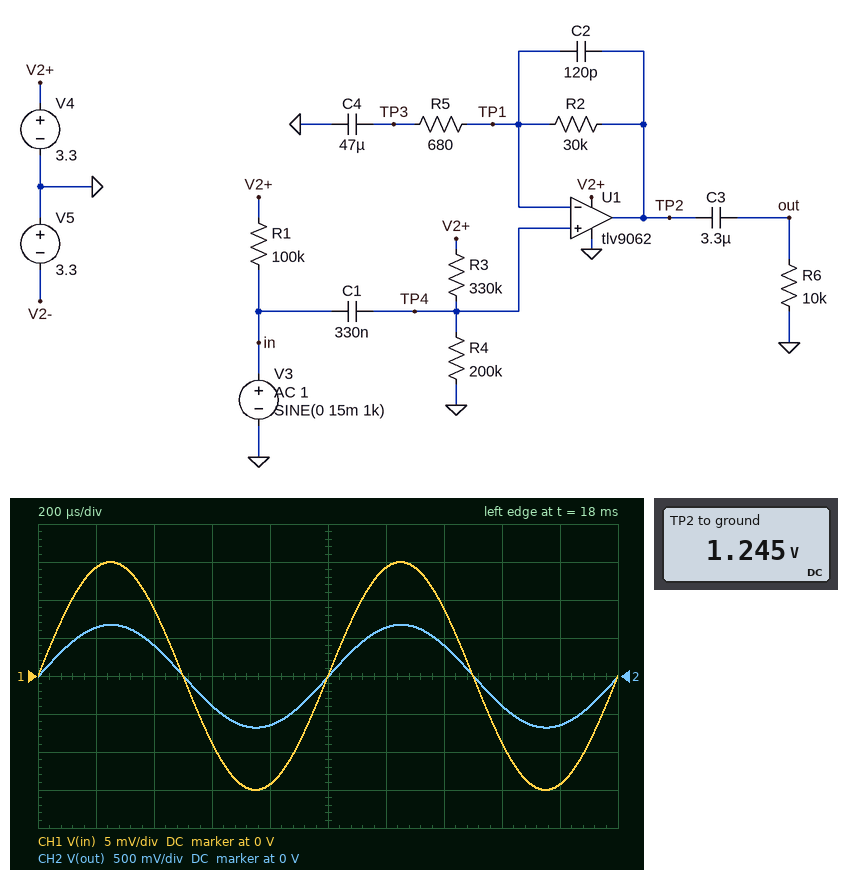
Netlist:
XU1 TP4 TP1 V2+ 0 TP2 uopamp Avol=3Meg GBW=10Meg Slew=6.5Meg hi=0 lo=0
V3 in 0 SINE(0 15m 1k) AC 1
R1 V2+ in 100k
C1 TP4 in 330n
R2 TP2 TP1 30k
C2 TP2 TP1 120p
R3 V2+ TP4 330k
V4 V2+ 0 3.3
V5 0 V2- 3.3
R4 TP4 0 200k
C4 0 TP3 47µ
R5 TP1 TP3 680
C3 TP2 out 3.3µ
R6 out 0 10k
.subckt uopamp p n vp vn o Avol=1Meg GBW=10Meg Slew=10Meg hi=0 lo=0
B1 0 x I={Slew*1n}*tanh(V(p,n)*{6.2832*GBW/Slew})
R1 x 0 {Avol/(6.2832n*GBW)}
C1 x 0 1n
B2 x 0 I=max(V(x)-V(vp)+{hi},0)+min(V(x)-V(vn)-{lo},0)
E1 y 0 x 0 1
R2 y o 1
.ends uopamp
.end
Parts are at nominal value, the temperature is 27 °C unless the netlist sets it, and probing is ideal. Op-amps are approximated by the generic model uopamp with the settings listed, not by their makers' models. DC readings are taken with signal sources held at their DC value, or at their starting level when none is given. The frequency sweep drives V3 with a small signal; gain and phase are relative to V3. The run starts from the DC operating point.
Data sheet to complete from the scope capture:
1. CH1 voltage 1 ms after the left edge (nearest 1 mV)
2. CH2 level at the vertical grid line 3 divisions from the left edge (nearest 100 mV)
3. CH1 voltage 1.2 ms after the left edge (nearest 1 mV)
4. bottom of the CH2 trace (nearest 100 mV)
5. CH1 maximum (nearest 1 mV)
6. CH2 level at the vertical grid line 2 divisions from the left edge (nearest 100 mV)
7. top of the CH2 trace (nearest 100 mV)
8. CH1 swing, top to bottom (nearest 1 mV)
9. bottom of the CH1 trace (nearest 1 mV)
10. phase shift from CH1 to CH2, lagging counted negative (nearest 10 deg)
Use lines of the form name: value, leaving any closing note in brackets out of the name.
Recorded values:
CH1 voltage 1 ms after the left edge: 0 V
CH2 level at the vertical grid line 3 divisions from the left edge: -400 mV
CH1 voltage 1.2 ms after the left edge: 14 mV
bottom of the CH2 trace: -700 mV
CH1 maximum: 15 mV
CH2 level at the vertical grid line 2 divisions from the left edge: 400 mV
top of the CH2 trace: 700 mV
CH1 swing, top to bottom: 30 mV
bottom of the CH1 trace: -15 mV
phase shift from CH1 to CH2, lagging counted negative: 0 deg
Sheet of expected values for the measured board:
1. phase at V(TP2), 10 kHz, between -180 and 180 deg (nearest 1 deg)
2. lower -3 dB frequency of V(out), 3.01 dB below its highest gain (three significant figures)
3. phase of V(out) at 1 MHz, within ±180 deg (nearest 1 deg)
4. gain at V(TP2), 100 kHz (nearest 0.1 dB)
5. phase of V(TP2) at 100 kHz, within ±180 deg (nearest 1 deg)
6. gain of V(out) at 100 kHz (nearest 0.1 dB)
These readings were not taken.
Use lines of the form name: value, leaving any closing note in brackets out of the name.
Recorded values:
phase at V(TP2), 10 kHz, between -180 and 180 deg: -15 deg
lower -3 dB frequency of V(out), 3.01 dB below its highest gain: 8.97 Hz
phase of V(out) at 1 MHz, within ±180 deg: -66 deg
gain at V(TP2), 100 kHz: 23.9 dB
phase of V(TP2) at 100 kHz, within ±180 deg: -67 deg
gain of V(out) at 100 kHz: 23.9 dB
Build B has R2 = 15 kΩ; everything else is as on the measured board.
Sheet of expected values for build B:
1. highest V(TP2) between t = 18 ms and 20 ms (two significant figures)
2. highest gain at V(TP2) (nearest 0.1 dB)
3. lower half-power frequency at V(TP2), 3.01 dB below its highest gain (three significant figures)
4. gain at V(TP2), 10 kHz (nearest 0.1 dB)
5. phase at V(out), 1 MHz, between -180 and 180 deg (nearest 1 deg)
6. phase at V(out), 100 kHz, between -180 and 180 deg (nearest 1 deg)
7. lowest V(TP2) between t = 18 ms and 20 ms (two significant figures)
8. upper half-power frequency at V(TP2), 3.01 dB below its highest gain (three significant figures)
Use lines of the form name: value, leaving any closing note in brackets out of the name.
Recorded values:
highest V(TP2) between t = 18 ms and 20 ms: 1.6 V
highest gain at V(TP2): 27.3 dB
lower half-power frequency at V(TP2), 3.01 dB below its highest gain: 6.89 Hz
gain at V(TP2), 10 kHz: 27.2 dB
phase at V(out), 1 MHz, between -180 and 180 deg: -64 deg
phase at V(out), 100 kHz, between -180 and 180 deg: -51 deg
lowest V(TP2) between t = 18 ms and 20 ms: 900 mV
upper half-power frequency at V(TP2), 3.01 dB below its highest gain: 74.0 kHz
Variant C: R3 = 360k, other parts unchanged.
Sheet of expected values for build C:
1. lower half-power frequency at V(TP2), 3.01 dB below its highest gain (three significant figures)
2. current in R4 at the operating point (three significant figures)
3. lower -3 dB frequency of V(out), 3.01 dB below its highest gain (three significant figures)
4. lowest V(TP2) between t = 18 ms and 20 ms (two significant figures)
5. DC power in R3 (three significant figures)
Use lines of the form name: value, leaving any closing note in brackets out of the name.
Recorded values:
lower half-power frequency at V(TP2), 3.01 dB below its highest gain: 6.81 Hz
current in R4 at the operating point: 5.89 µA
lower -3 dB frequency of V(out), 3.01 dB below its highest gain: 8.90 Hz
lowest V(TP2) between t = 18 ms and 20 ms: 500 mV
DC power in R3: 12.5 µW
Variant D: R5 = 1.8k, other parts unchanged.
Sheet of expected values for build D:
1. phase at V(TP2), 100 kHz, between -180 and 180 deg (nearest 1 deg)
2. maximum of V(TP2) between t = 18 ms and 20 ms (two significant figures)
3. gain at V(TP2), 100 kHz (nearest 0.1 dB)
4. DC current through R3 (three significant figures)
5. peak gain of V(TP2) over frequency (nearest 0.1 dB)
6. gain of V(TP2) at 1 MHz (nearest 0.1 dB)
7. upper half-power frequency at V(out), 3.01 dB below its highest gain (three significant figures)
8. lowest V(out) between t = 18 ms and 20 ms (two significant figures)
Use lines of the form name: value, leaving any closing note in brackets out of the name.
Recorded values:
phase at V(TP2), 100 kHz, between -180 and 180 deg: -61 deg
maximum of V(TP2) between t = 18 ms and 20 ms: 1.5 V
gain at V(TP2), 100 kHz: 16.6 dB
DC current through R3: 6.23 µA
peak gain of V(TP2) over frequency: 24.9 dB
gain of V(TP2) at 1 MHz: 1.4 dB
upper half-power frequency at V(out), 3.01 dB below its highest gain: 41.3 kHz
lowest V(out) between t = 18 ms and 20 ms: -270 mV
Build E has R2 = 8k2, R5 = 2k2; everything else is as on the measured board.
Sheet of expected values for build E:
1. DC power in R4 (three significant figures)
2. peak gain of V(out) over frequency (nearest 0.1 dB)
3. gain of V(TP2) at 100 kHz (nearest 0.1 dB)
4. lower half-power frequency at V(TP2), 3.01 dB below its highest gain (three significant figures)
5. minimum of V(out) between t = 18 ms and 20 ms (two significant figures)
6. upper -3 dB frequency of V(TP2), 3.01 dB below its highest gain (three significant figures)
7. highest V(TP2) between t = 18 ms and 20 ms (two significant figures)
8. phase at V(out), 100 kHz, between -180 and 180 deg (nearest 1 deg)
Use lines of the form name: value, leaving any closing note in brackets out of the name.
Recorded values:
DC power in R4: 7.75 µW
peak gain of V(out) over frequency: 13.5 dB
gain of V(TP2) at 100 kHz: 12.0 dB
lower half-power frequency at V(TP2), 3.01 dB below its highest gain: 4.36 Hz
minimum of V(out) between t = 18 ms and 20 ms: -71 mV
upper -3 dB frequency of V(TP2), 3.01 dB below its highest gain: 159 kHz
highest V(TP2) between t = 18 ms and 20 ms: 1.3 V
phase at V(out), 100 kHz, between -180 and 180 deg: -26 deg
